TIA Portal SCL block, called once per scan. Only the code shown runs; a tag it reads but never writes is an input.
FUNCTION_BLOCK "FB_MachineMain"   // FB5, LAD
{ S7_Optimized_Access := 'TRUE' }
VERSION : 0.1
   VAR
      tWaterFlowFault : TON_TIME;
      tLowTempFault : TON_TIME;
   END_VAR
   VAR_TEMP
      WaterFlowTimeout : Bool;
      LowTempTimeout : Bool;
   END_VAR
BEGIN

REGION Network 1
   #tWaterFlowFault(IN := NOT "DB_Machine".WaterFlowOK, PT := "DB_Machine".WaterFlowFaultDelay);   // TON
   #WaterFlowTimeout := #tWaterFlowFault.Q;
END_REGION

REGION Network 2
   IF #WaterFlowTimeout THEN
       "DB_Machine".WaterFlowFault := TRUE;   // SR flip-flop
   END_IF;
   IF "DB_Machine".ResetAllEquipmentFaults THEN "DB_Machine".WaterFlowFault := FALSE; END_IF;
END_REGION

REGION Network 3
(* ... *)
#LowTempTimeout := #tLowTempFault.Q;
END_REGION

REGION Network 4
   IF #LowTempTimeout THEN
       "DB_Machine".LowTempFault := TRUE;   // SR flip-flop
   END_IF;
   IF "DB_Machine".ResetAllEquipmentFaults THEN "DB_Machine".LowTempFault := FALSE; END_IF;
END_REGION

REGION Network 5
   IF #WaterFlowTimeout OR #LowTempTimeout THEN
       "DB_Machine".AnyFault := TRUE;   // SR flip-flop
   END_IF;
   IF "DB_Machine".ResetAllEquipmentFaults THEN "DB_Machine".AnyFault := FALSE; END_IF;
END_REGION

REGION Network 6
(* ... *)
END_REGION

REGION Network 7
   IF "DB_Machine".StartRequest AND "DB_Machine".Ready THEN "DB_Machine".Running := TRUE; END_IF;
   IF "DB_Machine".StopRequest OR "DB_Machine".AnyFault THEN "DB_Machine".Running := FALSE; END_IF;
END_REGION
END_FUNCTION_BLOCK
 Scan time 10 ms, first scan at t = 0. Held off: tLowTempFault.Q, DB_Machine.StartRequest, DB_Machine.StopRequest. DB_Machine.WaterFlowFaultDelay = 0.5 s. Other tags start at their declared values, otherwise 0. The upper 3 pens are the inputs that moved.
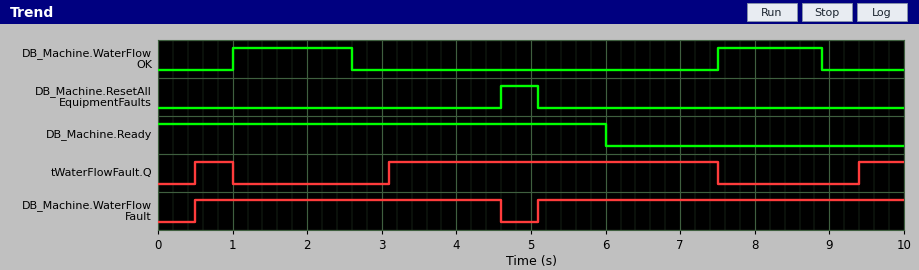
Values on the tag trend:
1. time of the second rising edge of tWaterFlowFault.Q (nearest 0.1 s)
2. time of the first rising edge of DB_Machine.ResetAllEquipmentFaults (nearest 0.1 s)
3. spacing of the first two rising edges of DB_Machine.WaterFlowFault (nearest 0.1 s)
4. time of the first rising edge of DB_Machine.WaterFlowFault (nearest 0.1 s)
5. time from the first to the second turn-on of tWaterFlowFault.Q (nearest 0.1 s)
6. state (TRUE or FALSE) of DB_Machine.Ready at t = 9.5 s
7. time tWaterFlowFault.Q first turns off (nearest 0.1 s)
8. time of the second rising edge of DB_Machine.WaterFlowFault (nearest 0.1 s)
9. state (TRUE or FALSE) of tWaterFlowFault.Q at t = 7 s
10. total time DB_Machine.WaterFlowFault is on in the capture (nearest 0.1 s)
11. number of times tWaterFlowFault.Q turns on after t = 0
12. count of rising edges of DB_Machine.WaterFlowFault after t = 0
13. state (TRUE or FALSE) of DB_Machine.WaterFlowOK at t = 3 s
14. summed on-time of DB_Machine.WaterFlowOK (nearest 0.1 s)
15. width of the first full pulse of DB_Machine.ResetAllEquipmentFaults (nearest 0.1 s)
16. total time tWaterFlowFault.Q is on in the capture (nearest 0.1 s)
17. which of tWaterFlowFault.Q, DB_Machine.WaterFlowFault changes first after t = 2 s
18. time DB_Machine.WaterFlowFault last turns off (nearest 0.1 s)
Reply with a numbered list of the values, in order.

1. 3.1 s
2. 4.6 s
3. 4.6 s
4. 0.5 s
5. 2.6 s
6. FALSE
7. 1.0 s
8. 5.1 s
9. TRUE
10. 9.0 s
11. 3
12. 2
13. FALSE
14. 3.0 s
15. 0.5 s
16. 5.5 s
17. tWaterFlowFault.Q
18. 4.6 s
